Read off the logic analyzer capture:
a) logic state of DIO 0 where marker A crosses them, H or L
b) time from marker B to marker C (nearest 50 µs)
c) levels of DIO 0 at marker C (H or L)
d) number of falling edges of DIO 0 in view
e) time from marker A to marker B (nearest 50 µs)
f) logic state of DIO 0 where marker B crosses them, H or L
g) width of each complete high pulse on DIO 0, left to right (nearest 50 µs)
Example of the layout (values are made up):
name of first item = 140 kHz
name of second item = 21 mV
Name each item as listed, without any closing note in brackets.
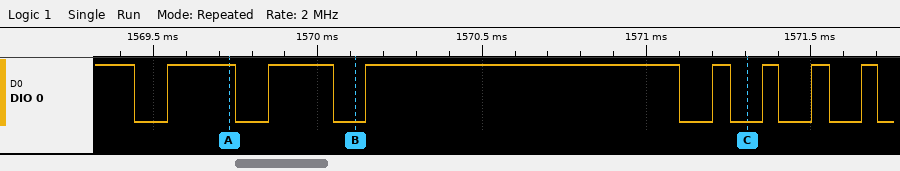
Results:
logic state of DIO 0 where marker A crosses them, H or L = DIO 0=H
time from marker B to marker C = 1200 µs
levels of DIO 0 at marker C = DIO 0=L
number of falling edges of DIO 0 in view = 8
time from marker A to marker B = 400 µs
logic state of DIO 0 where marker B crosses them, H or L = DIO 0=L
width of each complete high pulse on DIO 0, left to right = 200 µs, 200 µs, 950 µs, 50 µs, 50 µs, 50 µs, 50 µs
